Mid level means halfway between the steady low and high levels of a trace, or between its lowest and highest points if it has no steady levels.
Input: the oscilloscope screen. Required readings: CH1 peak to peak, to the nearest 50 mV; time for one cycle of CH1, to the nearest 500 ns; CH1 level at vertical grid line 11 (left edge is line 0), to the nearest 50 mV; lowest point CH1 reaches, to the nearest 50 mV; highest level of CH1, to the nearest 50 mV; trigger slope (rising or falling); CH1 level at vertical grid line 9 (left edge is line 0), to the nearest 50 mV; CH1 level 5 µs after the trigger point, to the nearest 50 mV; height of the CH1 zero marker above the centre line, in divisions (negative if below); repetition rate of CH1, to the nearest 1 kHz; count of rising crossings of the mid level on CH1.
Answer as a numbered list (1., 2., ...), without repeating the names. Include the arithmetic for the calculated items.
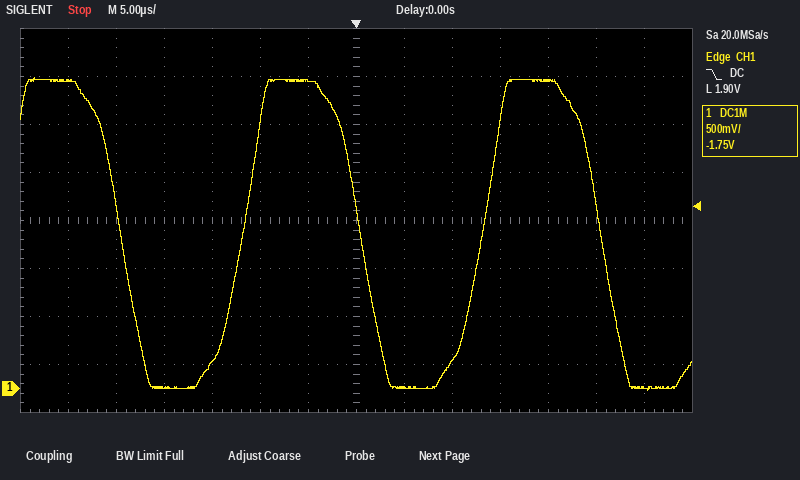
1. 3.25 V − (0 mV) = 3.25 V
2. 25.0 µs
3. 3.20 V
4. 0 mV
5. 3.25 V
6. falling
7. 300 mV
8. 0 mV
9. -3.5 div
10. 1 / 25.0 µs ≈ 40 kHz
11. 2
